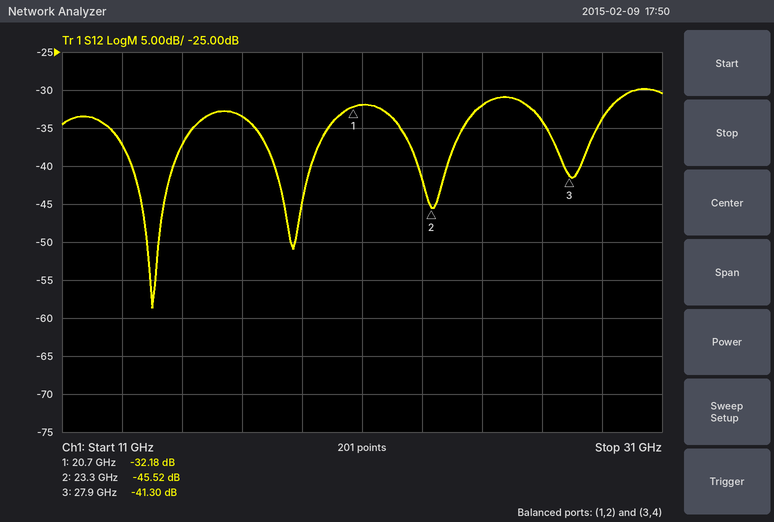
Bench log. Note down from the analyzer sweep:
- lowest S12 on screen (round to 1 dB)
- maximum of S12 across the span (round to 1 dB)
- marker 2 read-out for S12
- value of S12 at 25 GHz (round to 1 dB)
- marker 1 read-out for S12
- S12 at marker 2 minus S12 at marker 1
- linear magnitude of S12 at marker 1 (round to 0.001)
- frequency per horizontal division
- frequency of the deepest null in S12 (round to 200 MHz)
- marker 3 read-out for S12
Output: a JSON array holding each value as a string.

["-59 dB", "-30 dB", "-45.52 dB", "-32 dB", "-32.18 dB", "-13.34 dB", "0.025", "2 GHz", "14.0 GHz", "-41.30 dB"]
